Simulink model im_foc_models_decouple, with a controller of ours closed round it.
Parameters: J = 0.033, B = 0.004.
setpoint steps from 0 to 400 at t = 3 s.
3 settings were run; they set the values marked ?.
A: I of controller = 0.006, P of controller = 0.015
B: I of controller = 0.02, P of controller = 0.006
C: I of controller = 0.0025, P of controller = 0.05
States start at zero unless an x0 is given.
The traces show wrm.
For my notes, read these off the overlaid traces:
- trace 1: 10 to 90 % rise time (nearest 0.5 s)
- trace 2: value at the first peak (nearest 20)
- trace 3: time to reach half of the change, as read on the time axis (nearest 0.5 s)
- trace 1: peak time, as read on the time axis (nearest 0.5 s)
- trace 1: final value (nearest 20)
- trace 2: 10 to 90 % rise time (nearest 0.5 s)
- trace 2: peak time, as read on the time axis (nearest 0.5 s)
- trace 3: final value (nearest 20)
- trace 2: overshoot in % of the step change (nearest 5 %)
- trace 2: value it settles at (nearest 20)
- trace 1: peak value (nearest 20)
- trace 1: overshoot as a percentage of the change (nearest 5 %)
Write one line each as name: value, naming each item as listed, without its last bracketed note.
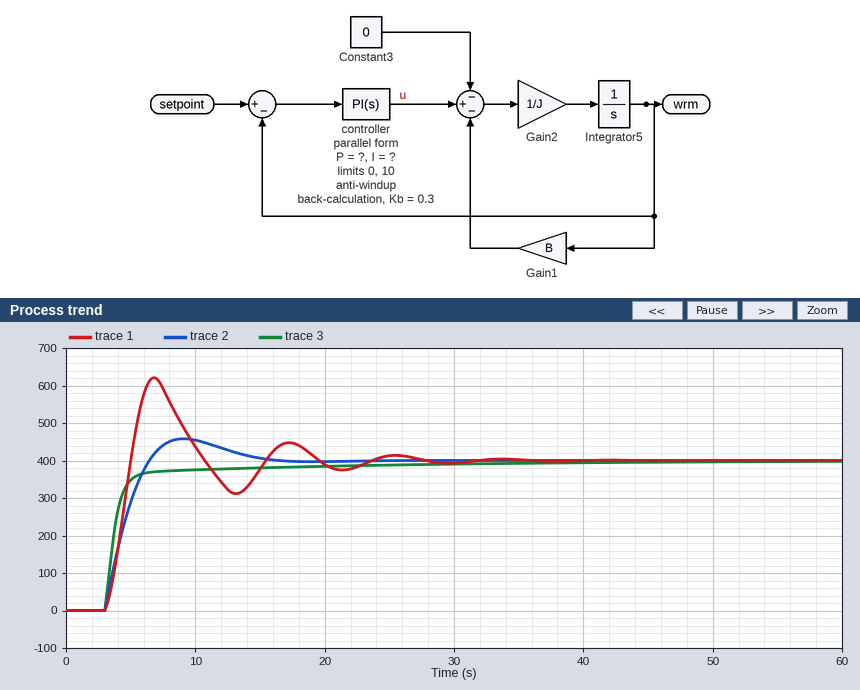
trace 1: 10 to 90 % rise time: 1.5 s
trace 2: value at the first peak: 460
trace 3: time to reach half of the change, as read on the time axis: 3.5 s
trace 1: peak time, as read on the time axis: 7.0 s
trace 1: final value: 400
trace 2: 10 to 90 % rise time: 2.5 s
trace 2: peak time, as read on the time axis: 9.0 s
trace 3: final value: 400
trace 2: overshoot in % of the step change: 15 %
trace 2: value it settles at: 400
trace 1: peak value: 620
trace 1: overshoot as a percentage of the change: 55 %
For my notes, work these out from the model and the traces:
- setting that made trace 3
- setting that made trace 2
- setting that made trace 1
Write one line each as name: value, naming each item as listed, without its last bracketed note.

setting that made trace 3: C
setting that made trace 2: A
setting that made trace 1: B
